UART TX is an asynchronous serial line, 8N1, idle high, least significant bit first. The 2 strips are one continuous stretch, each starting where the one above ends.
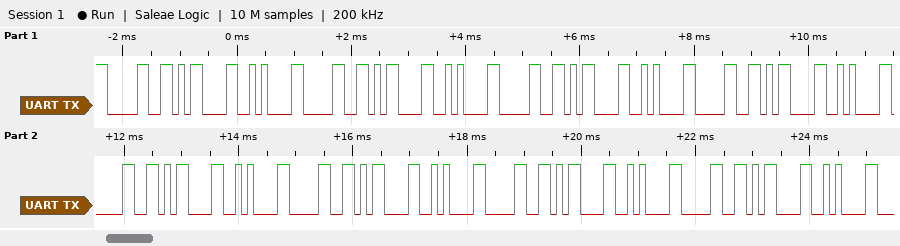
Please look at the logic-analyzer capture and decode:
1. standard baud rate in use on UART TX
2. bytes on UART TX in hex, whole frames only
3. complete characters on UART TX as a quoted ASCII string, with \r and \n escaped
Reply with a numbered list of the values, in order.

1. 9600 baud
2. 30 0D 0A 30 0D 0A 30 0D 0A 30 0D 0A 30 0D 0A 30 0D 0A 30 0D 0A 30 0D 0A
3. "0\r\n0\r\n0\r\n0\r\n0\r\n0\r\n0\r\n0\r\n"
